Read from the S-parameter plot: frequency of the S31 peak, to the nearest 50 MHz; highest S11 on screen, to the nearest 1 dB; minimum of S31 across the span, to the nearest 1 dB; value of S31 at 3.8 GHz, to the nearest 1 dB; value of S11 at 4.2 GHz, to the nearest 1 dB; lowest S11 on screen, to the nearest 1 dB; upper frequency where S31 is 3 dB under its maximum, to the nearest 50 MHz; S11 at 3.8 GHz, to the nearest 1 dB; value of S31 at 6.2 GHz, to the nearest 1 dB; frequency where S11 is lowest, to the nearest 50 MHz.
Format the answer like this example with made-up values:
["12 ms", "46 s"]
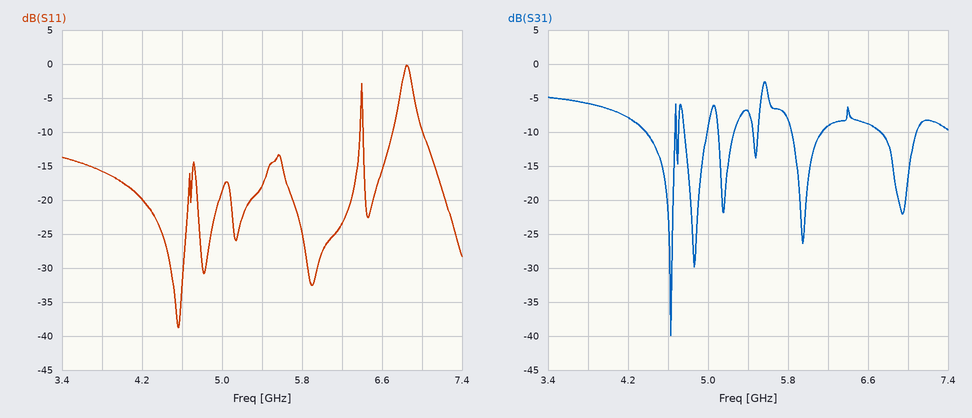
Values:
["5.55 GHz", "0 dB", "-40 dB", "-6 dB", "-20 dB", "-39 dB", "5.60 GHz", "-16 dB", "-9 dB", "4.55 GHz"]
